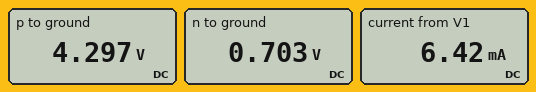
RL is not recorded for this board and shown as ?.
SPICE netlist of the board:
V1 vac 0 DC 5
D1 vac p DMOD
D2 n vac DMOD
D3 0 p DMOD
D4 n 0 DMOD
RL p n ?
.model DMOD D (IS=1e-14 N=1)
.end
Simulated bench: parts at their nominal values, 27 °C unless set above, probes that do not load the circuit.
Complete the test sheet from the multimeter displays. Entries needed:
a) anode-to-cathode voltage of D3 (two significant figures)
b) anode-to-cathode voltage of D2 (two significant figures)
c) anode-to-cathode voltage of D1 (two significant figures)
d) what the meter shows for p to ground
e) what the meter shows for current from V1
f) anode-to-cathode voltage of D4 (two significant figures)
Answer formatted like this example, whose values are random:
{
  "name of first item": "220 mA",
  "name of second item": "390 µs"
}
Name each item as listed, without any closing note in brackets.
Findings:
{
  "anode-to-cathode voltage of D3": "-4.3 V",
  "anode-to-cathode voltage of D2": "-4.3 V",
  "anode-to-cathode voltage of D1": "700 mV",
  "what the meter shows for p to ground": "4.297 V",
  "what the meter shows for current from V1": "6.42 mA",
  "anode-to-cathode voltage of D4": "700 mV"
}
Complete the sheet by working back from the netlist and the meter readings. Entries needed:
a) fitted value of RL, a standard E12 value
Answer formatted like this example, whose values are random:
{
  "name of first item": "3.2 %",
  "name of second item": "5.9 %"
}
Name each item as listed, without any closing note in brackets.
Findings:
{
  "fitted value of RL, a standard E12 value": "560 Ω"
}
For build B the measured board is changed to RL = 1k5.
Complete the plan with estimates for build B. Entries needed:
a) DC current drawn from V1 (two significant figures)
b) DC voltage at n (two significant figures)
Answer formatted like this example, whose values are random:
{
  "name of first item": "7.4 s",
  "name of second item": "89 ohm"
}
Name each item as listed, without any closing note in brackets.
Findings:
{
  "DC current drawn from V1": "2.4 mA",
  "DC voltage at n": "680 mV"
}
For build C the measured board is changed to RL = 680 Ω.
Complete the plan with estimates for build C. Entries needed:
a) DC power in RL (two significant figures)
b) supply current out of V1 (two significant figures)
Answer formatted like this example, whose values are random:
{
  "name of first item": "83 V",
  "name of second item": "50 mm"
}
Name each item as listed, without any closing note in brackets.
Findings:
{
  "DC power in RL": "19 mW",
  "supply current out of V1": "5.3 mA"
}
